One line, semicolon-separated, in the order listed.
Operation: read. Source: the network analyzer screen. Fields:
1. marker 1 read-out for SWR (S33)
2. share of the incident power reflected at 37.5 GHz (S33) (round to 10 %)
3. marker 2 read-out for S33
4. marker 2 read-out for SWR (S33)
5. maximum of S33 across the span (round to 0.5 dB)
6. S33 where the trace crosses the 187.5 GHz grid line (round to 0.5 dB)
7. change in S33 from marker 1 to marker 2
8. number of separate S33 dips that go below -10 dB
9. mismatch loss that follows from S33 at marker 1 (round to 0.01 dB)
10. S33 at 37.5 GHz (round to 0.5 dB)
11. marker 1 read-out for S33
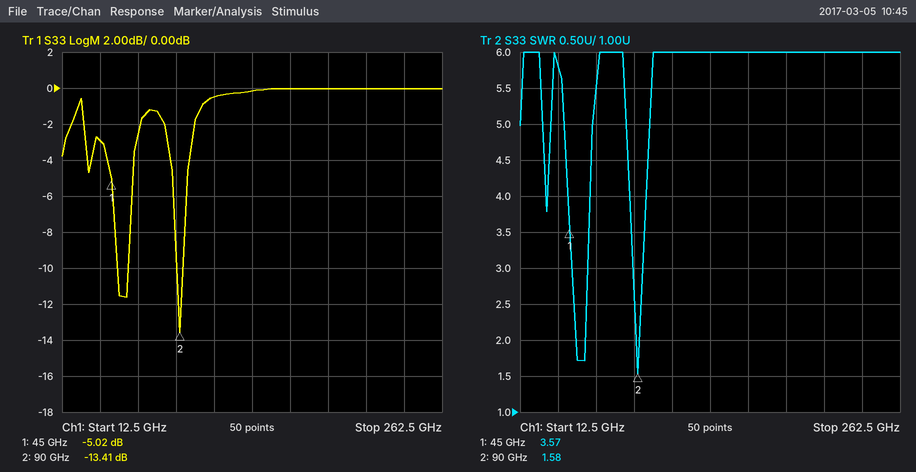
3.57; 50 %; -13.41 dB; 1.58; 0.0 dB; 0.0 dB; -8.39 dB; 2; 1.64 dB; -3.0 dB; -5.02 dB
